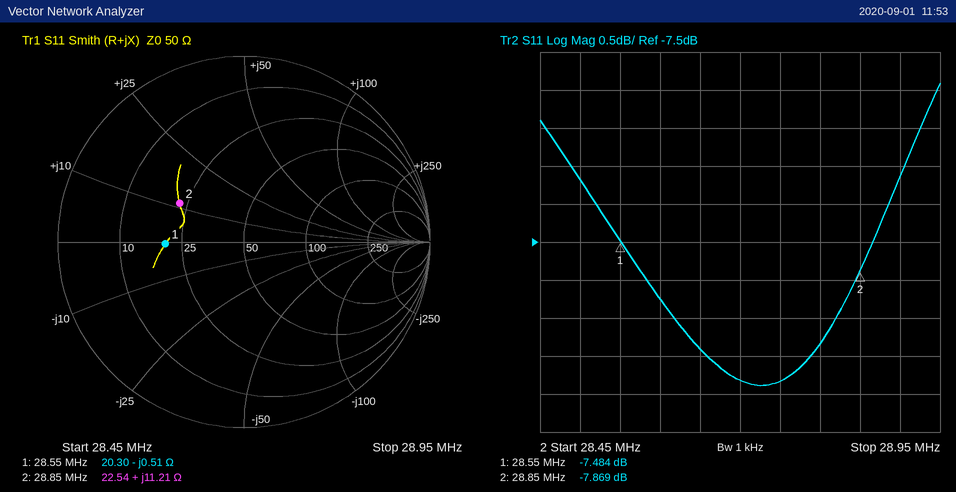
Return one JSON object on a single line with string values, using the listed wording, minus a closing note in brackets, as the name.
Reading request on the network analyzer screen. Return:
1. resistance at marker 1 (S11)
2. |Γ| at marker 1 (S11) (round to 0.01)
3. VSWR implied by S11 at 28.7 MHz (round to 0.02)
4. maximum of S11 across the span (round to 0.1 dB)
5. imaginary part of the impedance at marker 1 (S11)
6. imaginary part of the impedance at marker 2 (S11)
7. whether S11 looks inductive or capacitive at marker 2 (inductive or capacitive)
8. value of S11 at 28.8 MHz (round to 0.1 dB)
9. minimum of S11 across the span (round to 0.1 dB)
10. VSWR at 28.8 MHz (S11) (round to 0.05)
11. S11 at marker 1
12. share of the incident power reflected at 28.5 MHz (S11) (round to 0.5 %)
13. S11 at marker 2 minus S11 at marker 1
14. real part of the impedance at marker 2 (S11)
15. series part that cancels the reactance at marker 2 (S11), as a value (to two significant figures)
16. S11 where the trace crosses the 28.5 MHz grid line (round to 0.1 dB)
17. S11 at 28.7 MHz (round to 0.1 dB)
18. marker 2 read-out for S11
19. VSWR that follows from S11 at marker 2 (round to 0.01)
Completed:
{"resistance at marker 1": "20.30 Ω", "|Γ| at marker 1 (S11)": "0.42", "VSWR implied by S11 at 28.7 MHz": "2.04", "maximum of S11 across the span": "-5.4 dB", "imaginary part of the impedance at marker 1": "-0.51 Ω", "imaginary part of the impedance at marker 2": "+11.21 Ω", "whether S11 looks inductive or capacitive at marker 2": "inductive", "value of S11 at 28.8 MHz": "-8.8 dB", "minimum of S11 across the span": "-9.4 dB", "VSWR at 28.8 MHz (S11)": "2.15", "S11 at marker 1": "-7.484 dB", "share of the incident power reflected at 28.5 MHz (S11)": "21.5 %", "S11 at marker 2 minus S11 at marker 1": "-0.385 dB", "real part of the impedance at marker 2": "22.54 Ω", "series part that cancels the reactance at marker 2 (S11), as a value": "490 pF", "S11 where the trace crosses the 28.5 MHz grid line": "-6.7 dB", "S11 at 28.7 MHz": "-9.3 dB", "marker 2 read-out for S11": "-7.869 dB", "VSWR that follows from S11 at marker 2": "2.36"}
